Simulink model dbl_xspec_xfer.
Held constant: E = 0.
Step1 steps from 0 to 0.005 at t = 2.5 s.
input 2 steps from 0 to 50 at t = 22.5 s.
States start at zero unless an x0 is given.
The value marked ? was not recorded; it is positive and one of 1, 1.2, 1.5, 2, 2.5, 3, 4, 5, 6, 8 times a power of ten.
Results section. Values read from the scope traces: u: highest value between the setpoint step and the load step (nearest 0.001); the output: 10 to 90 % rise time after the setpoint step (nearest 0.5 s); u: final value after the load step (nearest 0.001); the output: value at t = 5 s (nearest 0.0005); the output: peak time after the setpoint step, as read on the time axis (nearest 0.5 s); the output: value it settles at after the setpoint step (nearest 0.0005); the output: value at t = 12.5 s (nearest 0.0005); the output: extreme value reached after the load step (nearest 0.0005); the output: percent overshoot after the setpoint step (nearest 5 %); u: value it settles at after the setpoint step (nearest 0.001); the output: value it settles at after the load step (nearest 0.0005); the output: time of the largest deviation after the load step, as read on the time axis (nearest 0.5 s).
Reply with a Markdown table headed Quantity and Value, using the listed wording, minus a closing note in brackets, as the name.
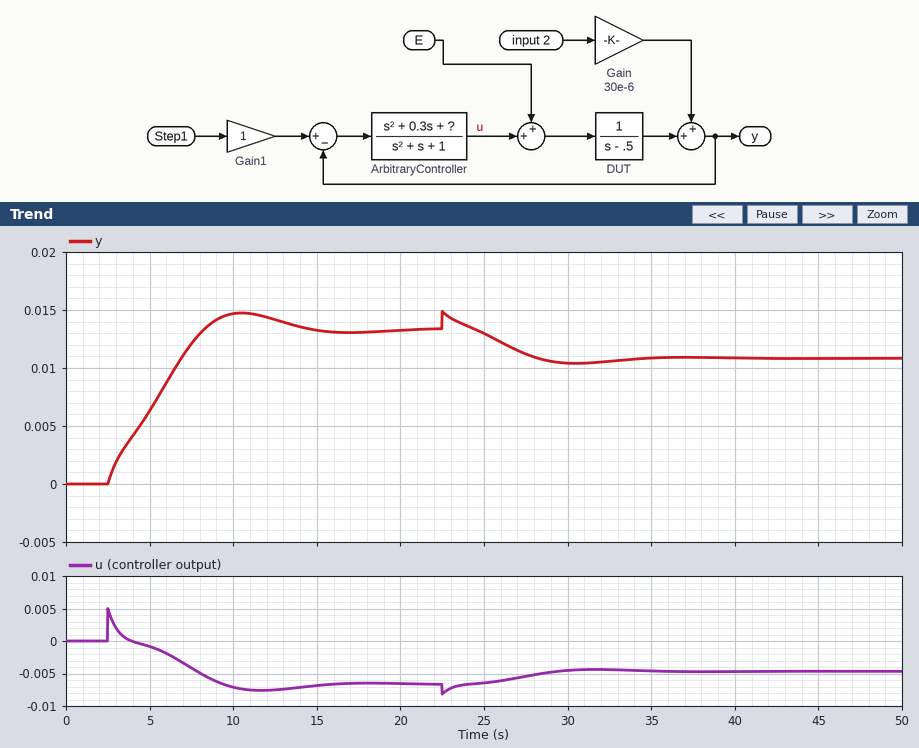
| Quantity | Value |
|---|---|
| u: highest value between the setpoint step and the load step | 0.005 |
| the output: 10 to 90 % rise time after the setpoint step | 4.5 s |
| u: final value after the load step | -0.005 |
| the output: value at t = 5 s | 0.0065 |
| the output: peak time after the setpoint step, as read on the time axis | 10.5 s |
| the output: value it settles at after the setpoint step | 0.0135 |
| the output: value at t = 12.5 s | 0.0140 |
| the output: extreme value reached after the load step | 0.0105 |
| the output: percent overshoot after the setpoint step | 10 % |
| u: value it settles at after the setpoint step | -0.007 |
| the output: value it settles at after the load step | 0.0110 |
| the output: time of the largest deviation after the load step, as read on the time axis | 30.5 s |
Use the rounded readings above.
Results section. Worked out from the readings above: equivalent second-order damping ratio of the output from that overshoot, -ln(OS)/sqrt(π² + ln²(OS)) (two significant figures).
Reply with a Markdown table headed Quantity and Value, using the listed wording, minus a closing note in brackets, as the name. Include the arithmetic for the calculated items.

| Quantity | Value |
|---|---|
| equivalent second-order damping ratio of the output from that overshoot, -ln(OS)/sqrt(π² + ln²(OS)) | ln(0.1) = -2.303; 2.303 / sqrt(9.870 + 5.302) = 0.59 |
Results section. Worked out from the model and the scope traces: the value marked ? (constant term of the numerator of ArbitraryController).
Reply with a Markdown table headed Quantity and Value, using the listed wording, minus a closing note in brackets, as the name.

| Quantity | Value |
|---|---|
| the value marked ? | 0.8 |
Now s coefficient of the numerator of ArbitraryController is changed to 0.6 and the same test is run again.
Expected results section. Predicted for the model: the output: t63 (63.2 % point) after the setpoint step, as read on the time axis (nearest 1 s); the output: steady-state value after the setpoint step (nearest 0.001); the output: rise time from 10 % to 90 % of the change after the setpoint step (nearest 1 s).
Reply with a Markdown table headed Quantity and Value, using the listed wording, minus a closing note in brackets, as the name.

| Quantity | Value |
|---|---|
| the output: t63 (63.2 % point) after the setpoint step, as read on the time axis | 6 s |
| the output: steady-state value after the setpoint step | 0.013 |
| the output: rise time from 10 % to 90 % of the change after the setpoint step | 6 s |
